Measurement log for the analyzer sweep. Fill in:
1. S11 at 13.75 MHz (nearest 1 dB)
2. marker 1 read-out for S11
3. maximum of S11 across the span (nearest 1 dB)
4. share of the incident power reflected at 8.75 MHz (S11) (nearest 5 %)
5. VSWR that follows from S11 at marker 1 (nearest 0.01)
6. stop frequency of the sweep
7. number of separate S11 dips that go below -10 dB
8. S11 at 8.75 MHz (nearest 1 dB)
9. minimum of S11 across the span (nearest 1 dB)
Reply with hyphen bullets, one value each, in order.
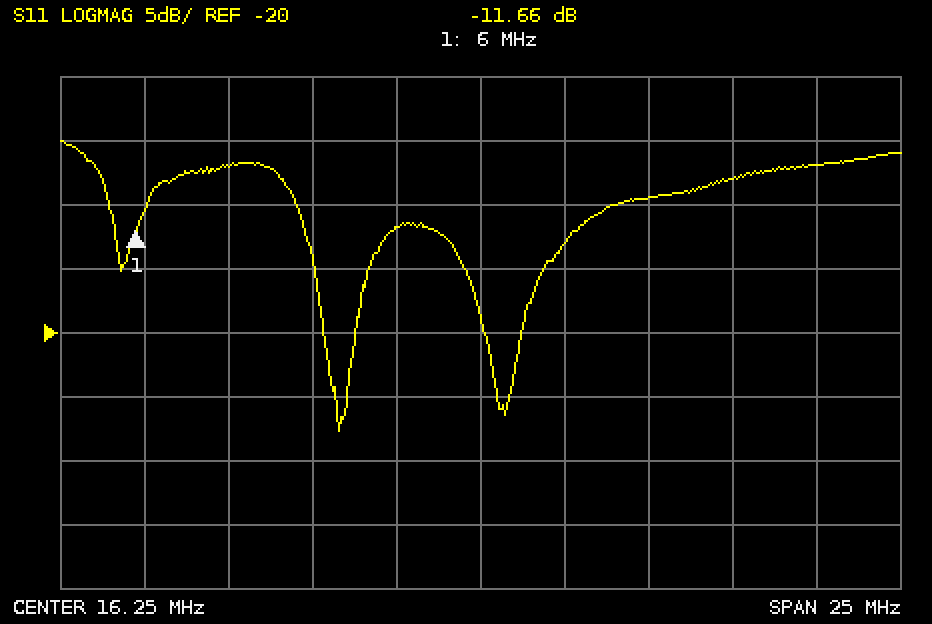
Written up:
- -12 dB
- -11.66 dB
- -5 dB
- 20 %
- 1.71
- 28.75 MHz
- 3
- -7 dB
- -28 dB
